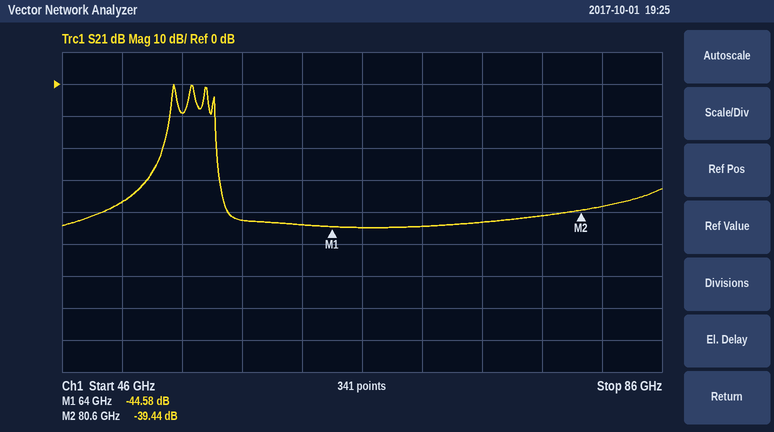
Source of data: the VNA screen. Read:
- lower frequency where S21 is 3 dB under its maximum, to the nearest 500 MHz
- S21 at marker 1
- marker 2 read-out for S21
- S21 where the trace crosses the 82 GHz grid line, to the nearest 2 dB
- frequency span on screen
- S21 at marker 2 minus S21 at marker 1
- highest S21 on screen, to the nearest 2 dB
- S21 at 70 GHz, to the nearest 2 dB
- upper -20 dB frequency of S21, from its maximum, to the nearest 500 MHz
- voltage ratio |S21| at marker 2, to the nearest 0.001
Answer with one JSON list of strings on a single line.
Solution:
["53.5 GHz", "-44.58 dB", "-39.44 dB", "-38 dB", "40 GHz", "5.14 dB", "0 dB", "-44 dB", "56.5 GHz", "0.011"]
